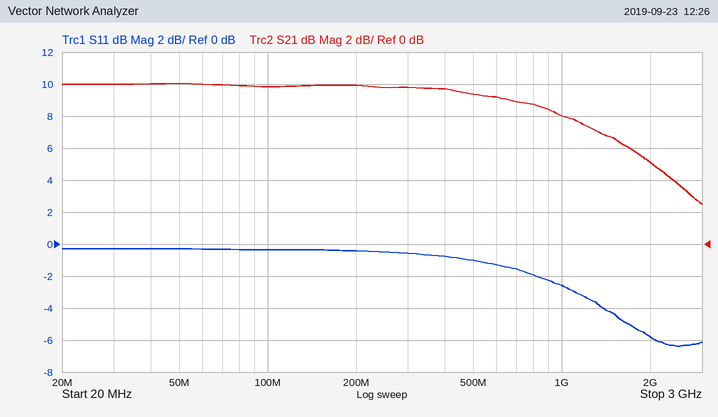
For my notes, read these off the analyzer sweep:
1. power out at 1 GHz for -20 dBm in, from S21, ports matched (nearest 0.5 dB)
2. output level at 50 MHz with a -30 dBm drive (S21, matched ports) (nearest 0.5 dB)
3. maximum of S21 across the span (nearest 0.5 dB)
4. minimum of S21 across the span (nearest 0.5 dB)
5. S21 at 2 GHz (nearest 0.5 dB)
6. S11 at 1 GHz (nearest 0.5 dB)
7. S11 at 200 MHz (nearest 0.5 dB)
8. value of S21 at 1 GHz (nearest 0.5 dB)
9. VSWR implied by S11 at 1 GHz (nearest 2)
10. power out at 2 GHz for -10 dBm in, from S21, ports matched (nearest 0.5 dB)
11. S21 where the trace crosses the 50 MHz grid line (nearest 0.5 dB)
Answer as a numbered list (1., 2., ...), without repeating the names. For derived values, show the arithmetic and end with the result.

1. -20 dBm + (8.0 dB) = -12.0 dBm
2. -30 dBm + (10.0 dB) = -20.0 dBm
3. 10.0 dB
4. 2.5 dB
5. 5.0 dB
6. -2.5 dB
7. -0.5 dB
8. 8.0 dB
9. |Γ| = 10^(-2.5/20) = 0.7499; VSWR = (1 + 0.7499)/(1 − 0.7499) ≈ 7.00, so 6 to the nearest 2
10. -10 dBm + (5.0 dB) = -5.0 dBm
11. 10.0 dB
